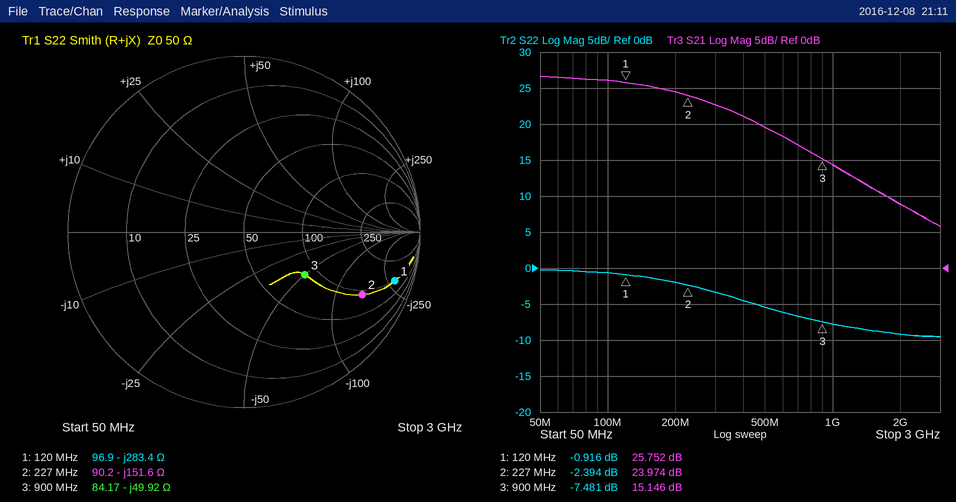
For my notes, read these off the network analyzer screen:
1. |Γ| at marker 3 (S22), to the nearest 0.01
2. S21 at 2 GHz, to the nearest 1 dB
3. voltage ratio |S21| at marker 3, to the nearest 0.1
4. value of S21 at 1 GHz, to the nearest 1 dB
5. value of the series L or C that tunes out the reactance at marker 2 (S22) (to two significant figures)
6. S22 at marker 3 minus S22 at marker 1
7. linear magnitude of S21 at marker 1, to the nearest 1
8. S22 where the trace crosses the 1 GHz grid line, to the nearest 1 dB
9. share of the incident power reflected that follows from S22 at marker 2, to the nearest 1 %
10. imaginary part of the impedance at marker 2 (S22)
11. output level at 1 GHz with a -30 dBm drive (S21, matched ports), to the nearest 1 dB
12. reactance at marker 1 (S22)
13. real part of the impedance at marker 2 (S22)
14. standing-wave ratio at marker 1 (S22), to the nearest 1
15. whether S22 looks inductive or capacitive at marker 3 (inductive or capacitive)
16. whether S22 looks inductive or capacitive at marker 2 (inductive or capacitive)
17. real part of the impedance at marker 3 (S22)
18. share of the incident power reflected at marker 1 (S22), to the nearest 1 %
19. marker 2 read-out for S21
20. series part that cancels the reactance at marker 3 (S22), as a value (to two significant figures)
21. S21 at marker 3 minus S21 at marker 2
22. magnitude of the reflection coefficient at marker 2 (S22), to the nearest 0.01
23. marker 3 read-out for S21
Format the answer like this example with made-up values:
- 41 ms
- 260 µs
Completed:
- 0.42
- 9 dB
- 5.7
- 14 dB
- 110 nH
- -6.565 dB
- 19
- -8 dB
- 58 %
- -151.6 Ω
- -16 dBm
- -283.4 Ω
- 90.2 Ω
- 19
- capacitive
- capacitive
- 84.17 Ω
- 81 %
- 23.974 dB
- 8.8 nH
- -8.828 dB
- 0.76
- 15.146 dB
